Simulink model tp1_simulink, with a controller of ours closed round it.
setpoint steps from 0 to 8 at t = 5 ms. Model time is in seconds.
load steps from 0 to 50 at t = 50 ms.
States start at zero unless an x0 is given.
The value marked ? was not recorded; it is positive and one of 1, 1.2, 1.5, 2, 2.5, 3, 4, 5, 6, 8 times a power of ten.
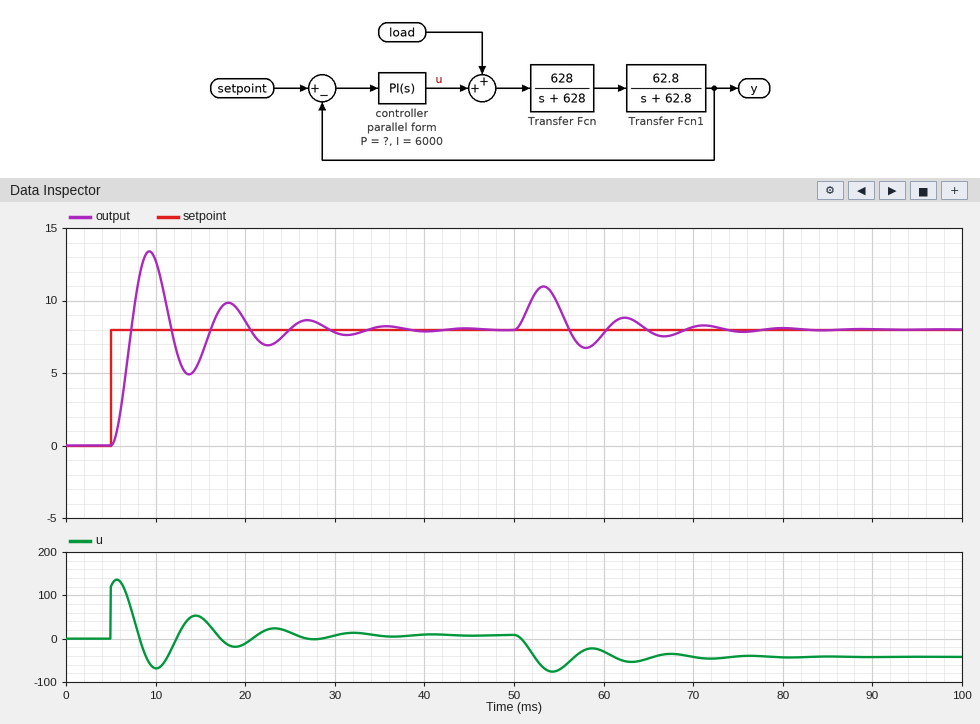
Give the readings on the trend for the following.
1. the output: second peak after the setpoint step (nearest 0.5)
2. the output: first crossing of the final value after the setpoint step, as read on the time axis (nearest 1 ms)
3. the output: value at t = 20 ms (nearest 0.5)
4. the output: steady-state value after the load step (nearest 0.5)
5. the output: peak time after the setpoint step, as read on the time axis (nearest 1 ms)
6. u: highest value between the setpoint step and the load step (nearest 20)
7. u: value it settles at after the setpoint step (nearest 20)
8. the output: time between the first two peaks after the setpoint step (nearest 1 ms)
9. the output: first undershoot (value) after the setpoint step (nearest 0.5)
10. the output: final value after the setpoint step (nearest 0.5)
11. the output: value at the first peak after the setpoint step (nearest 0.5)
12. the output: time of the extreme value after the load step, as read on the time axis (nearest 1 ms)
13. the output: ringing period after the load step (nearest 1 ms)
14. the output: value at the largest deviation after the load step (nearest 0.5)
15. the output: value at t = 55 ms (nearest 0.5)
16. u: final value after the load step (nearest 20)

10.0
7 ms
8.5
8.0
9 ms
140
0
9 ms
5.0
8.0
13.5
53 ms
9 ms
11.0
9.5
-40
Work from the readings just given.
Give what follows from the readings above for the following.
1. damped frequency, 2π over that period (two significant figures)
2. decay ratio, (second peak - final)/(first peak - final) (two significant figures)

0.70 rad/ms
0.36
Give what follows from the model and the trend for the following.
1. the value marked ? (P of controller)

15
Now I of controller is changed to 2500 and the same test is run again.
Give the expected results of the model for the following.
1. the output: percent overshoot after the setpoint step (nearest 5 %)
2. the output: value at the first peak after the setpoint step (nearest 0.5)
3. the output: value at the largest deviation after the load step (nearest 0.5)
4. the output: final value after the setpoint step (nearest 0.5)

40 %
11.0
11.5
8.0
